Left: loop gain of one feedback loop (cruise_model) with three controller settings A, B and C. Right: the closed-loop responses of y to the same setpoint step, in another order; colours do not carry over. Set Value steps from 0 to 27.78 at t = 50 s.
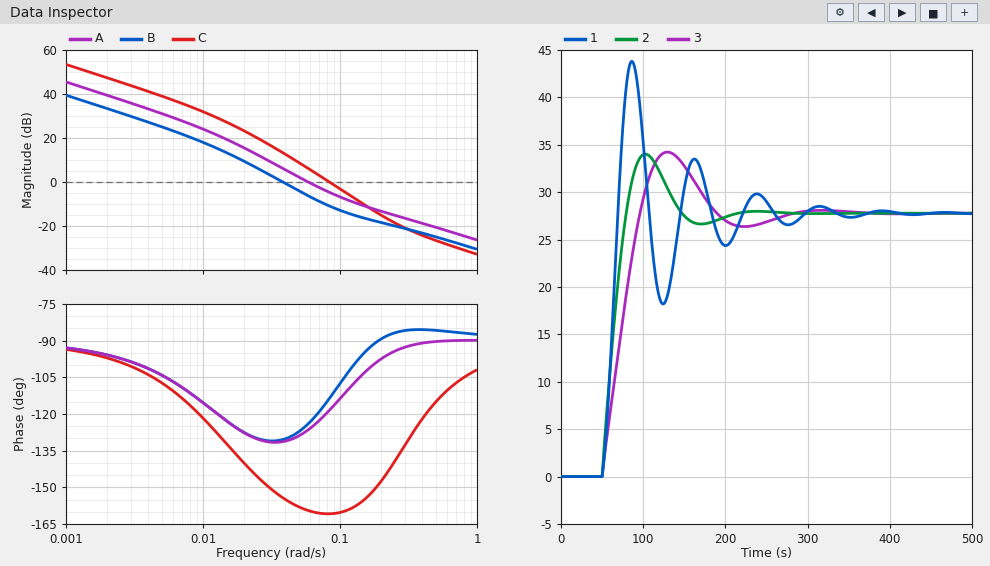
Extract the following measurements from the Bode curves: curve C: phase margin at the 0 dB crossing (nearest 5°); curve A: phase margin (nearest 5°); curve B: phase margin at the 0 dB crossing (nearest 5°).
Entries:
20°
55°
50°
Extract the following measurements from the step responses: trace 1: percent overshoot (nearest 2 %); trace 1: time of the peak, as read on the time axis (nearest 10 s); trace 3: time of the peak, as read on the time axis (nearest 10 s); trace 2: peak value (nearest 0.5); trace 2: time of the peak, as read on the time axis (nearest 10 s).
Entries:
58 %
90 s
130 s
34.0
100 s
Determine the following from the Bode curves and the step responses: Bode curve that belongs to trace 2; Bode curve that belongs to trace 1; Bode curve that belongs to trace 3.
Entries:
A
C
B
